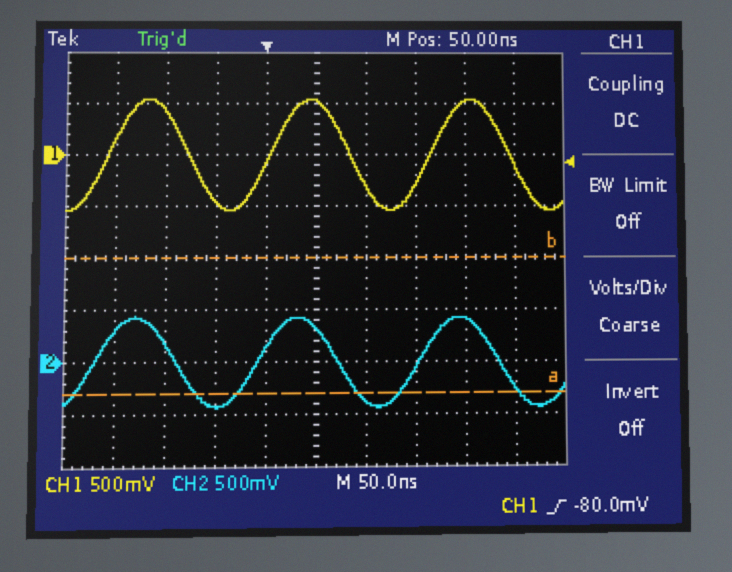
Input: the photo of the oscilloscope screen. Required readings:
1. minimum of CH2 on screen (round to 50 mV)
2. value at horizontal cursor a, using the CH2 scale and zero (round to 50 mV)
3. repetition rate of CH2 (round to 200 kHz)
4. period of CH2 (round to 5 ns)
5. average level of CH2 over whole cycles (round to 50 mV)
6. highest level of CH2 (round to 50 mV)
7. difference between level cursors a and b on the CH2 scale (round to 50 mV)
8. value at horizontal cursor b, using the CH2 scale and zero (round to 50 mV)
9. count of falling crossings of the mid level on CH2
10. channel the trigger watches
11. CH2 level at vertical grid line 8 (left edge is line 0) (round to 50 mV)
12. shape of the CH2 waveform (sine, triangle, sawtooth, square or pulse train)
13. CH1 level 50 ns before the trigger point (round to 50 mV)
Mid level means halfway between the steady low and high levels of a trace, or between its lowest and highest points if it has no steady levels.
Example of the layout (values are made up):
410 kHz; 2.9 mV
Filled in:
-450 mV; -300 mV; 6.2 MHz; 160 ns; 0 mV; 450 mV; 1.30 V; 1.00 V; 3; CH1; 400 mV; sine; -450 mV
